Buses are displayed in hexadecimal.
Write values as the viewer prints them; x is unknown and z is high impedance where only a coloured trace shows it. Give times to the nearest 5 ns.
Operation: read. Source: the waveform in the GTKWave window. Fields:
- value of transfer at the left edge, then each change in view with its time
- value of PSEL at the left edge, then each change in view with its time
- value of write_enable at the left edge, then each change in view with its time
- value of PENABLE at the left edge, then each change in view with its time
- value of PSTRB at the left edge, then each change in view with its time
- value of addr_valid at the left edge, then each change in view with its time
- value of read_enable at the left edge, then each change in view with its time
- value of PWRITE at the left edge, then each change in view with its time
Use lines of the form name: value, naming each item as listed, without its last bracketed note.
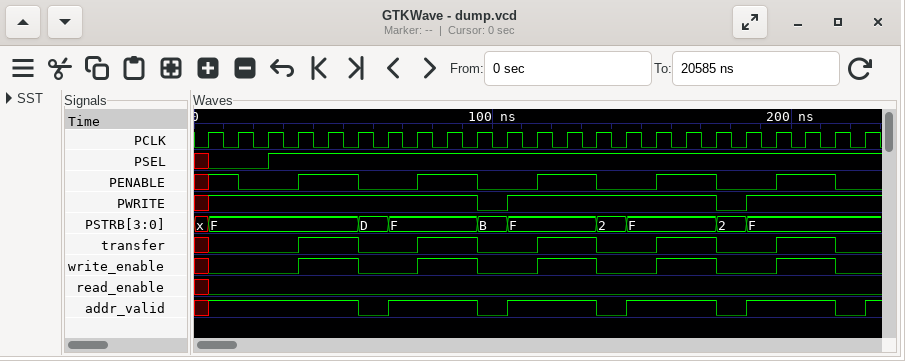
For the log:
value of transfer at the left edge, then each change in view with its time: x, 0 at 5 ns, 1 at 35 ns, 0 at 55 ns, 1 at 75 ns, 0 at 95 ns, 1 at 115 ns, 0 at 135 ns, 1 at 155 ns, 0 at 175 ns, 1 at 195 ns, 0 at 215 ns
value of PSEL at the left edge, then each change in view with its time: x, 0 at 5 ns, 1 at 25 ns
value of write_enable at the left edge, then each change in view with its time: x, 0 at 5 ns, 1 at 35 ns, 0 at 55 ns, 1 at 75 ns, 0 at 95 ns, 1 at 115 ns, 0 at 135 ns, 1 at 155 ns, 0 at 175 ns, 1 at 195 ns, 0 at 215 ns
value of PENABLE at the left edge, then each change in view with its time: x, 1 at 5 ns, 0 at 15 ns, 1 at 35 ns, 0 at 55 ns, 1 at 75 ns, 0 at 95 ns, 1 at 115 ns, 0 at 135 ns, 1 at 155 ns, 0 at 175 ns, 1 at 195 ns, 0 at 215 ns
value of PSTRB at the left edge, then each change in view with its time: x, F at 5 ns, D at 55 ns, F at 65 ns, B at 95 ns, F at 105 ns, 2 at 135 ns, F at 145 ns, 2 at 175 ns, F at 185 ns
value of addr_valid at the left edge, then each change in view with its time: x, 1 at 5 ns, 0 at 55 ns, 1 at 65 ns, 0 at 95 ns, 1 at 105 ns, 0 at 135 ns, 1 at 145 ns, 0 at 175 ns, 1 at 185 ns, 0 at 215 ns, 1 at 225 ns
value of read_enable at the left edge, then each change in view with its time: x, 0 at 5 ns
value of PWRITE at the left edge, then each change in view with its time: x, 1 at 5 ns, 0 at 95 ns, 1 at 105 ns, 0 at 175 ns, 1 at 185 ns
